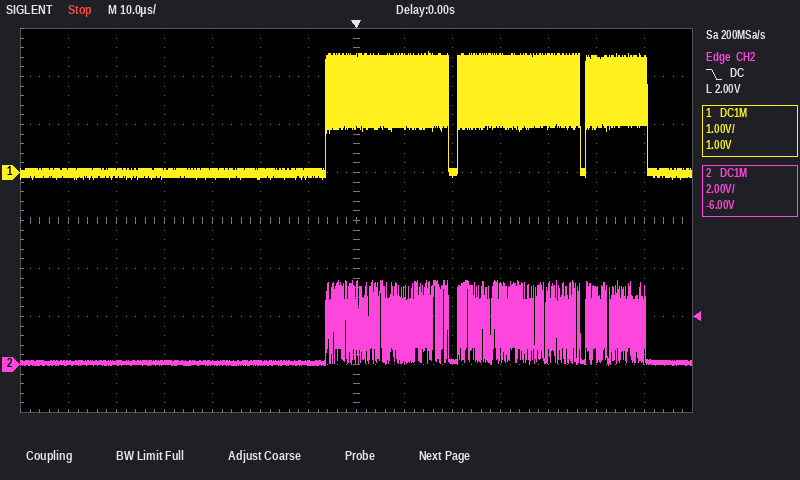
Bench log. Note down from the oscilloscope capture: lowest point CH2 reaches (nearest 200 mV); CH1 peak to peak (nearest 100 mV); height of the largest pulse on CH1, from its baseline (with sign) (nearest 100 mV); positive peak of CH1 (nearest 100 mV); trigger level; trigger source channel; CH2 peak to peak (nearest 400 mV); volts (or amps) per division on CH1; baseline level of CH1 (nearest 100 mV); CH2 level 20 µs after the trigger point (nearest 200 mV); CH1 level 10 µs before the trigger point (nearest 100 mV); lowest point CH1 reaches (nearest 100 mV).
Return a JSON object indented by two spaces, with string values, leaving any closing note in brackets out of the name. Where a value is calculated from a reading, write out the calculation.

{
  "lowest point CH2 reaches": "0.0 V",
  "CH1 peak to peak": "2.5 V − (-100 mV) = 2.6 V",
  "height of the largest pulse on CH1, from its baseline (with sign)": "2.5 V − (0.0 V) = +2.5 V",
  "positive peak of CH1": "2.5 V",
  "trigger level": "2.00 V",
  "trigger source channel": "CH2",
  "CH2 peak to peak": "3.6 V",
  "volts (or amps) per division on CH1": "1 V",
  "baseline level of CH1": "0.0 V",
  "CH2 level 20 µs after the trigger point": "200 mV",
  "CH1 level 10 µs before the trigger point": "0.0 V",
  "lowest point CH1 reaches": "-100 mV"
}
